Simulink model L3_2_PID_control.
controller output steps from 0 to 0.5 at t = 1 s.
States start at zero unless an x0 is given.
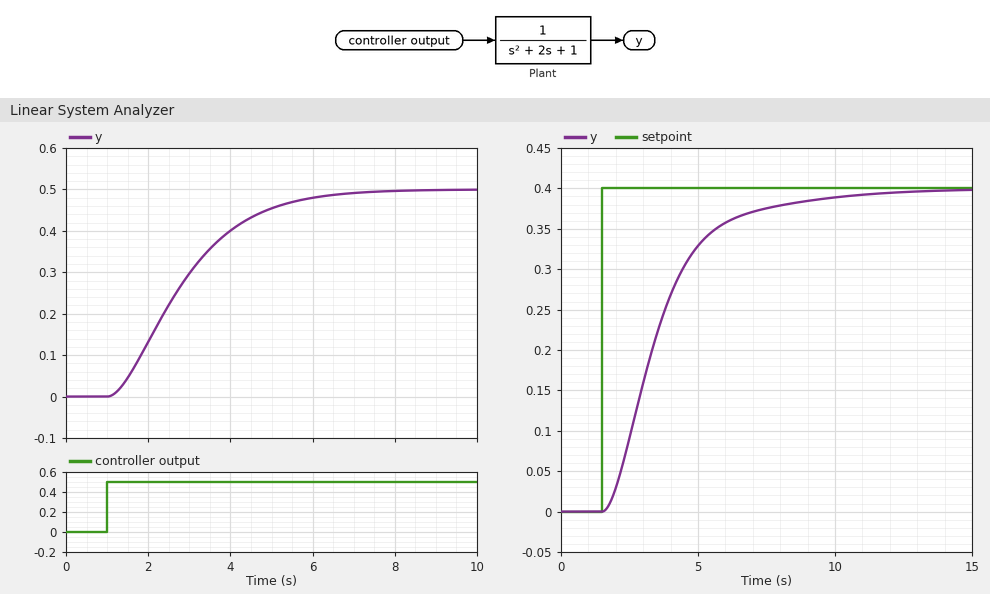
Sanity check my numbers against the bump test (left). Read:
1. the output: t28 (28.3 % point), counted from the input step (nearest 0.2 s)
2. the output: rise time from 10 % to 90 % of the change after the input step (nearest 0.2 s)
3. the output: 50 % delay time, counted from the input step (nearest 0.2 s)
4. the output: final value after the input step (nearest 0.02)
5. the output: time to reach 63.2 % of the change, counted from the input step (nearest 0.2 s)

1.0 s
3.4 s
1.6 s
0.50
2.2 s
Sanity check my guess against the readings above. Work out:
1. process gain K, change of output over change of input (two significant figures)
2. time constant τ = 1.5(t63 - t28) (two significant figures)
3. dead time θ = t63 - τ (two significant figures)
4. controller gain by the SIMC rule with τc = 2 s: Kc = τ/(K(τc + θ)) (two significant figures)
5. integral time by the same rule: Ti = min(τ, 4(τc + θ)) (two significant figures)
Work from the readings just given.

1.0
1.8 s
0.40 s
0.75
1.8 s
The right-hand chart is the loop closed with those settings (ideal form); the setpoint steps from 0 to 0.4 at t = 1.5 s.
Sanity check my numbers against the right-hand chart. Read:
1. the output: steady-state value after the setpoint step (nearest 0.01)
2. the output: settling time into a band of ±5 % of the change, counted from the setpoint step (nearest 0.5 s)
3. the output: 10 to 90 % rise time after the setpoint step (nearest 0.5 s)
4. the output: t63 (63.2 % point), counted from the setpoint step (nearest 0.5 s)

0.40
6.5 s
4.0 s
2.5 s
